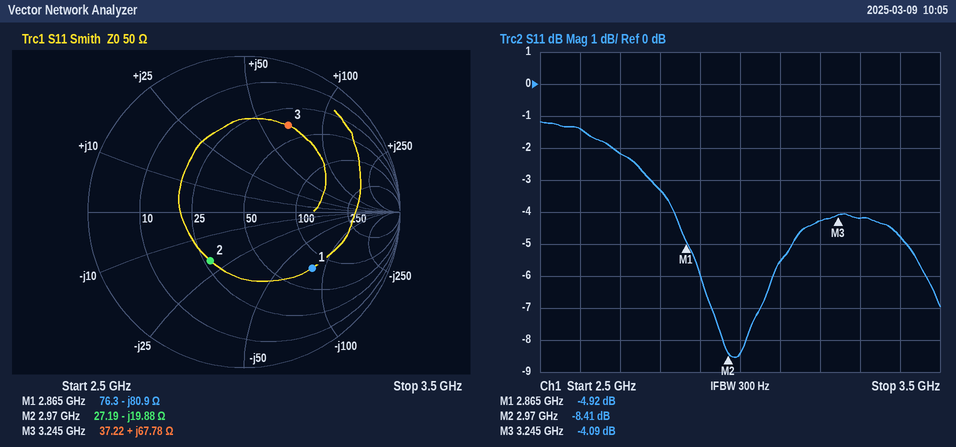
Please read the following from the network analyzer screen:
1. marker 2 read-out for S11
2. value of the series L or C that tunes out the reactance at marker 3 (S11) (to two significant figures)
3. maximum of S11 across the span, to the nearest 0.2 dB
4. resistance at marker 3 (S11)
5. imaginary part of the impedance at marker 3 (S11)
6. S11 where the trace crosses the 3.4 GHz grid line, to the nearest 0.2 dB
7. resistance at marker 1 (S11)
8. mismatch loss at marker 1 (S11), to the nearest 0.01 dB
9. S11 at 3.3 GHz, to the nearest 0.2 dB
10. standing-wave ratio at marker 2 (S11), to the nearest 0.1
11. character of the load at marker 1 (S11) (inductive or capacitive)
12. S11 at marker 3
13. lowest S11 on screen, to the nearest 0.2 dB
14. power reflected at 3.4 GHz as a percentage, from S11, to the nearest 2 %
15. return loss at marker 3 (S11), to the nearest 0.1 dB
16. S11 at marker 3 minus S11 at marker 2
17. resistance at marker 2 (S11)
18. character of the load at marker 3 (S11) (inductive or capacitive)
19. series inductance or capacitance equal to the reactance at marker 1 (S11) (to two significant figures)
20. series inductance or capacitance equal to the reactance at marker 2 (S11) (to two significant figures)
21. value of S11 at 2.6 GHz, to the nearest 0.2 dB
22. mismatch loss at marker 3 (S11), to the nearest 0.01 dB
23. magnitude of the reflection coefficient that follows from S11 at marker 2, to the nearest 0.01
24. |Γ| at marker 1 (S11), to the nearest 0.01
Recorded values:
-8.41 dB
720 fF
-1.2 dB
37.22 Ω
+67.78 Ω
-4.8 dB
76.3 Ω
1.69 dB
-4.2 dB
2.2
capacitive
-4.09 dB
-8.6 dB
34 %
4.1 dB
4.32 dB
27.19 Ω
inductive
690 fF
2.7 pF
-1.4 dB
2.15 dB
0.38
0.57
